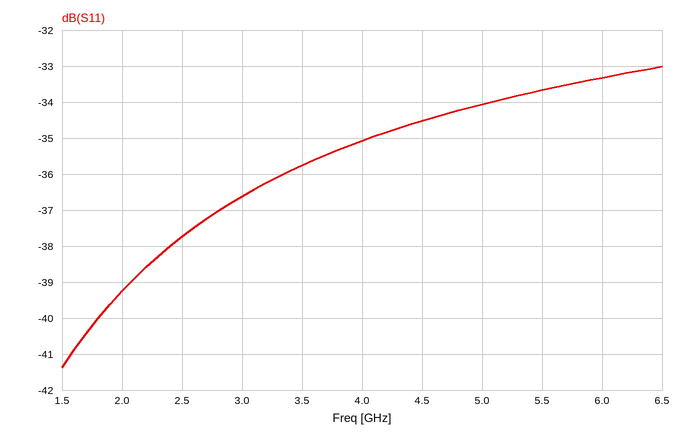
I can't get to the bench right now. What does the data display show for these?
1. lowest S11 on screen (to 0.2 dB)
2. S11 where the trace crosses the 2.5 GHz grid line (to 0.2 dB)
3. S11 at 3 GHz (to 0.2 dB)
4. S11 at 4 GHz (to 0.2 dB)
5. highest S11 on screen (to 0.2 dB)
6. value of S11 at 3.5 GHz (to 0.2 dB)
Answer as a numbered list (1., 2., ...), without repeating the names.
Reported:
1. -41.4 dB
2. -37.8 dB
3. -36.6 dB
4. -35.0 dB
5. -33.0 dB
6. -35.8 dB
